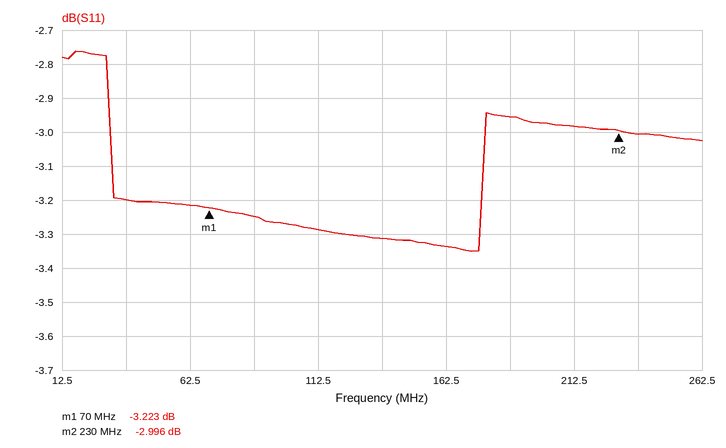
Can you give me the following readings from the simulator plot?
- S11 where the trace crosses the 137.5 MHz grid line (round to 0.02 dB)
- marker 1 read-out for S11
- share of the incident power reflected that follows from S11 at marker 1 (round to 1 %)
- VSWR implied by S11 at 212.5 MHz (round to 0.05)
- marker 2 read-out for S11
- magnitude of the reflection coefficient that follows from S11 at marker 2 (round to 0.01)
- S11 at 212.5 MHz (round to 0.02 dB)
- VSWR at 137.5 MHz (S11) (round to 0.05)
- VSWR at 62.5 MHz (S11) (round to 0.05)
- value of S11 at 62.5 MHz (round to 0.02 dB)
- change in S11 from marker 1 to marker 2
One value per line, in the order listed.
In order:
-3.32 dB
-3.223 dB
48 %
5.90
-2.996 dB
0.71
-2.98 dB
5.30
5.45
-3.22 dB
0.227 dB
